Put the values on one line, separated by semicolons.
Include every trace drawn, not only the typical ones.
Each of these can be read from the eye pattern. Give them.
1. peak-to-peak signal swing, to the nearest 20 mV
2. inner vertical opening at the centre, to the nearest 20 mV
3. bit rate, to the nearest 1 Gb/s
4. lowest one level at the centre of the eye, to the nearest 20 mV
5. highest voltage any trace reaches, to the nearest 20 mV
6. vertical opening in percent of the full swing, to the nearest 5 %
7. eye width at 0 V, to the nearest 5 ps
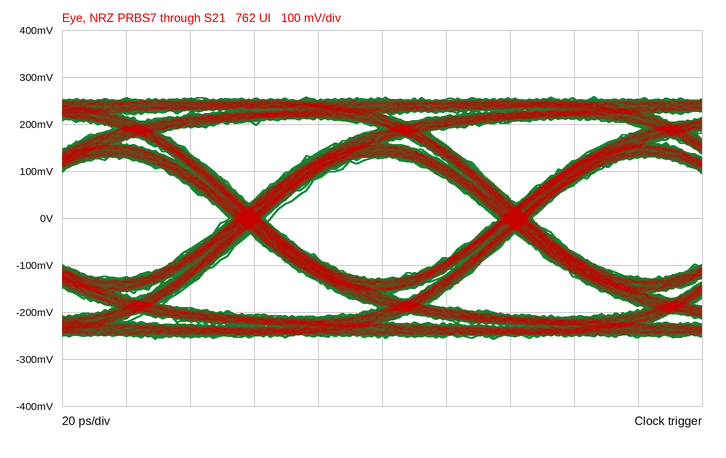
520 mV; 260 mV; 12 Gb/s; 120 mV; 260 mV; 50 %; 70 ps
